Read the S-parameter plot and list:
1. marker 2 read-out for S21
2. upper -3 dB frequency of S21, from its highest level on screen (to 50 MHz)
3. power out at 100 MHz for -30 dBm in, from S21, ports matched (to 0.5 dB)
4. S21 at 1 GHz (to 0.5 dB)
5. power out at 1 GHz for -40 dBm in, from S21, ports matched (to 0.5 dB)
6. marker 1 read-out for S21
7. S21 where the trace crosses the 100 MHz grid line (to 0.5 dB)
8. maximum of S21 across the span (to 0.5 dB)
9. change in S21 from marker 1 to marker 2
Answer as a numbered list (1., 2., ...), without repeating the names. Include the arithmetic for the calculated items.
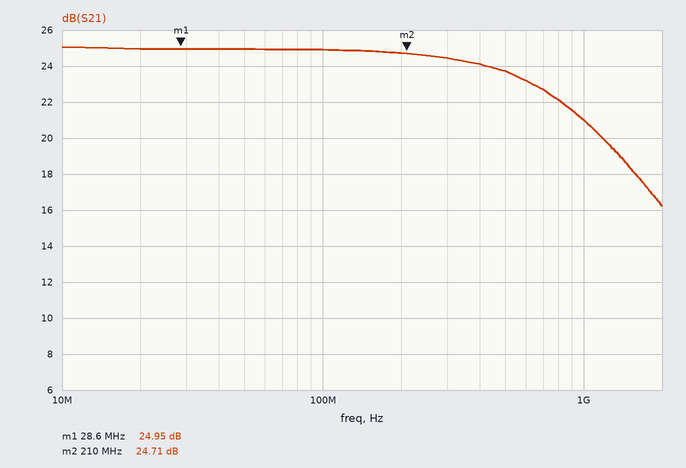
1. 24.71 dB
2. 800 MHz
3. -30 dBm + (25.0 dB) = -5.0 dBm
4. 21.0 dB
5. -40 dBm + (21.0 dB) = -19.0 dBm
6. 24.95 dB
7. 25.0 dB
8. 25.0 dB
9. 24.71 − (24.95) = -0.24 dB
